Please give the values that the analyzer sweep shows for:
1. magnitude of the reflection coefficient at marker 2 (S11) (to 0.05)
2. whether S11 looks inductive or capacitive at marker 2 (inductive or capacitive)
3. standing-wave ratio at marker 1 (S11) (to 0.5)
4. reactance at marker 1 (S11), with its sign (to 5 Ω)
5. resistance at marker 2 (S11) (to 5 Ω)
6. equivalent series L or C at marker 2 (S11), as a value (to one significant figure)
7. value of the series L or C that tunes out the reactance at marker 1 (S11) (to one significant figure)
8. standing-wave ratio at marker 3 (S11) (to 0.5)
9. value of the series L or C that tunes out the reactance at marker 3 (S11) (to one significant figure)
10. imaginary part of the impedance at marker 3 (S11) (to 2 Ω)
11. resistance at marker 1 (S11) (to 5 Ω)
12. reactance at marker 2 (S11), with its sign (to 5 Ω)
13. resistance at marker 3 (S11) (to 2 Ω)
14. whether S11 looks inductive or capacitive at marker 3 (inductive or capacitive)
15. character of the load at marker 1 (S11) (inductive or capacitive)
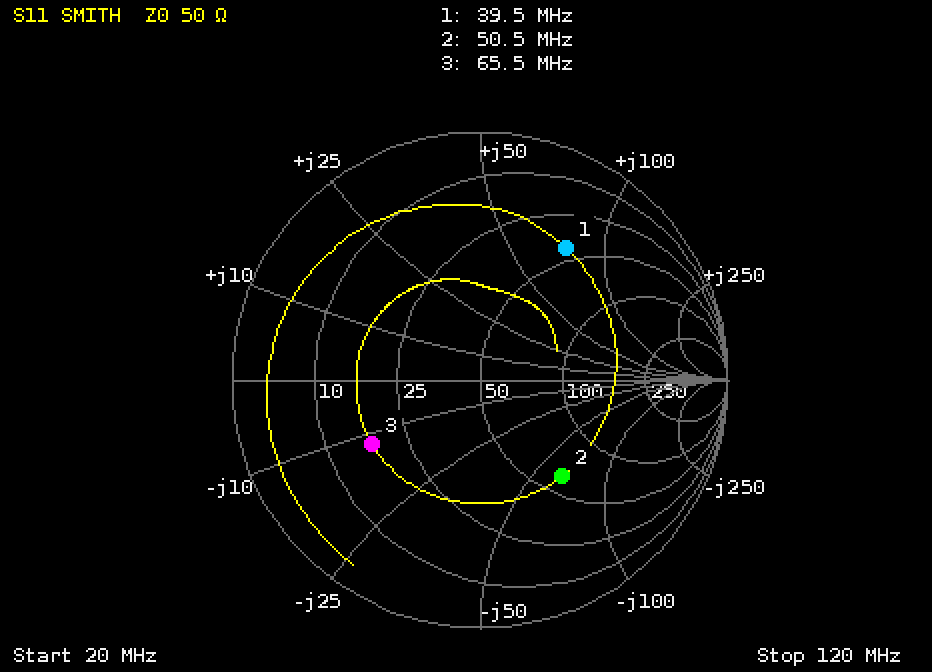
0.50
capacitive
4.5
+75 Ω
60 Ω
50 pF
50 pF
3.0
30 nH
-12 Ω
40 Ω
-65 Ω
18 Ω
capacitive
inductive
